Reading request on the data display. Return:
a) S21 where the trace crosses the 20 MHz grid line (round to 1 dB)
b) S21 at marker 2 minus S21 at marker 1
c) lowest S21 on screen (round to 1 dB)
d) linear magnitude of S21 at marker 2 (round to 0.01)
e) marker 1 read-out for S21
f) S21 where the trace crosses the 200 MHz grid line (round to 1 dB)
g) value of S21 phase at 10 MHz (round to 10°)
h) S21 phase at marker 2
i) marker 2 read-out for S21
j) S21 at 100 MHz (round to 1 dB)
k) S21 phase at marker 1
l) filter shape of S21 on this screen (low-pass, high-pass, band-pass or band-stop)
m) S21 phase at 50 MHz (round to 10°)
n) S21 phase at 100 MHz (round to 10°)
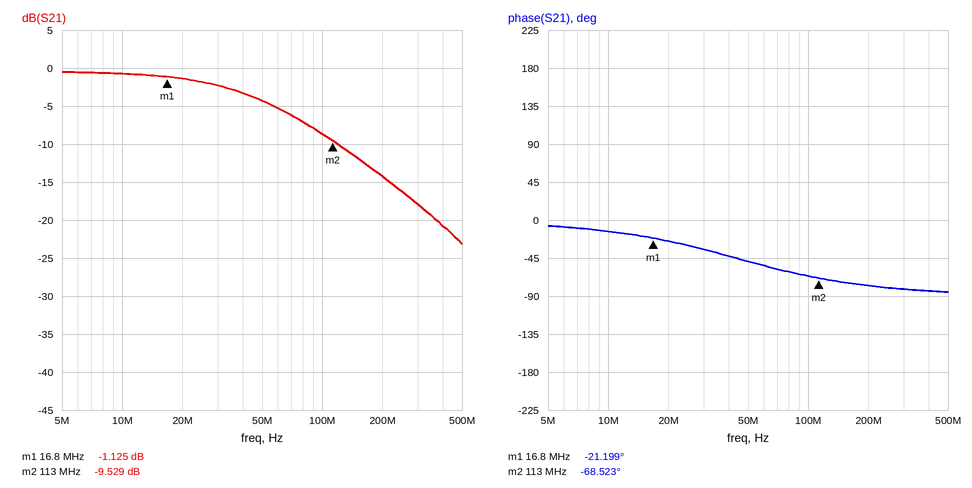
-1 dB
-8.404 dB
-23 dB
0.33
-1.125 dB
-14 dB
-10°
-68.523°
-9.529 dB
-9 dB
-21.199°
low-pass
-50°
-70°
